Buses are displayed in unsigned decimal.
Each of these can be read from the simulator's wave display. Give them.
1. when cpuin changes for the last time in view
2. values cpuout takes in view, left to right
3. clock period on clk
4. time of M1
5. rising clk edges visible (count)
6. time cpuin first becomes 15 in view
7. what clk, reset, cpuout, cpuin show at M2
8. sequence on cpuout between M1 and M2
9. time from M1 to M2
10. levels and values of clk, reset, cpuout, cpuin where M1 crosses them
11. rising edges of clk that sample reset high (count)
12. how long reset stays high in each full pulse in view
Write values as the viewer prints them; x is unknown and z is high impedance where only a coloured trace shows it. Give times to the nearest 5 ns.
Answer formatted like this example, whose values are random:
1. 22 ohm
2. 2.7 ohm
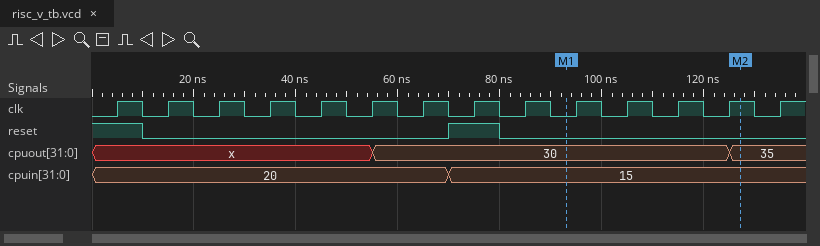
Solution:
1. 70 ns
2. x, 30, 35
3. 10 ns
4. 95 ns
5. 14
6. 70 ns
7. clk=1, reset=0, cpuout=35, cpuin=15
8. 30, 35
9. 35 ns
10. clk=0, reset=0, cpuout=30, cpuin=15
11. 2
12. 10 ns
